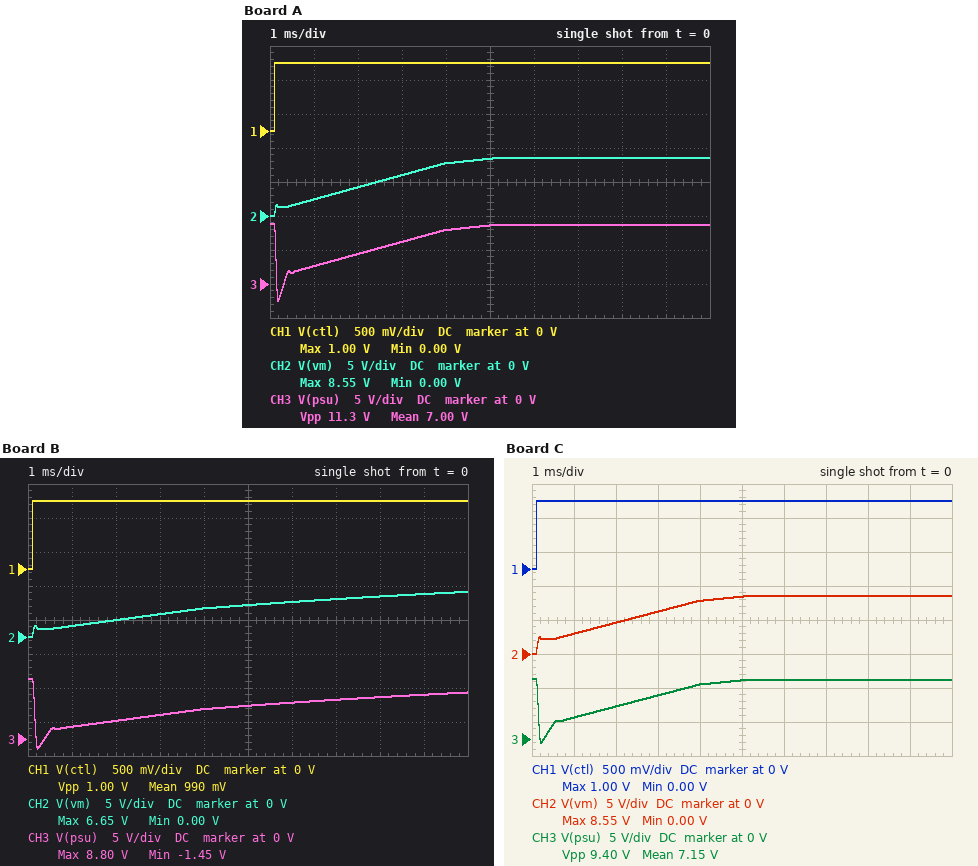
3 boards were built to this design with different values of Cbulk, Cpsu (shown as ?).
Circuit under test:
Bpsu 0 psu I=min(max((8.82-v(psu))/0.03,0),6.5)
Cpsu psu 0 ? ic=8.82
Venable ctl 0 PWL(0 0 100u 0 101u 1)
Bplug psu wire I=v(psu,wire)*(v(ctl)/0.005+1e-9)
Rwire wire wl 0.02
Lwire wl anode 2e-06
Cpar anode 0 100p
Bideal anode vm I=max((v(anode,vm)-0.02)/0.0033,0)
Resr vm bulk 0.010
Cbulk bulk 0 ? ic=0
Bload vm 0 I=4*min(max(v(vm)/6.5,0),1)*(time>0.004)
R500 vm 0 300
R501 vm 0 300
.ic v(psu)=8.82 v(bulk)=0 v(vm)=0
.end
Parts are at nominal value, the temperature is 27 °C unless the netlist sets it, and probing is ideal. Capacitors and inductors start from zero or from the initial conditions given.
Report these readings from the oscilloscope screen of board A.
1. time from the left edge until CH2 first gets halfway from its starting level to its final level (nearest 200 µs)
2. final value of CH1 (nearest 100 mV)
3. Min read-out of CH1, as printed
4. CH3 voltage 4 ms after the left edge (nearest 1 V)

2.0 ms
1.0 V
0.00 V
8 V
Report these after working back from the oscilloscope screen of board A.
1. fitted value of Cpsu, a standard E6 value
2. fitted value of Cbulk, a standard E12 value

330 µF
3.3 mF
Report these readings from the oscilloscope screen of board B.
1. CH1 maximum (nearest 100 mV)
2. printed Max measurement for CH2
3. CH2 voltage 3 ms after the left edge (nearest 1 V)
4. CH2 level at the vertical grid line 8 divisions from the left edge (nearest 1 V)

1.0 V
6.65 V
3 V
6 V
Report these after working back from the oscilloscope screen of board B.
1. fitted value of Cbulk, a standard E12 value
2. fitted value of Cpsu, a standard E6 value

6.8 mF
680 µF
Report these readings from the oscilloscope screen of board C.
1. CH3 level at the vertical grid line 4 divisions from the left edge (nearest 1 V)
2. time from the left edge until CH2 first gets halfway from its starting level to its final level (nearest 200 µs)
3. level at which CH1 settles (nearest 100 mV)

8 V
1.8 ms
1.0 V
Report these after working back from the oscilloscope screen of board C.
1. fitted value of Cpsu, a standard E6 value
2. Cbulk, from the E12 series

680 µF
3.3 mF
